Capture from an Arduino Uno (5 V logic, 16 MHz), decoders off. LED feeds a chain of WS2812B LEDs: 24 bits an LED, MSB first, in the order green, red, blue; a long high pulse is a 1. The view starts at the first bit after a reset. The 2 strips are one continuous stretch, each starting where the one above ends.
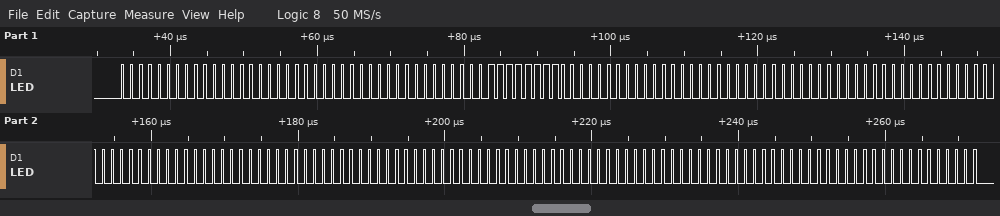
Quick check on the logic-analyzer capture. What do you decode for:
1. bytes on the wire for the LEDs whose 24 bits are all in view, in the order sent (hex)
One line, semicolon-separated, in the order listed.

00 00 00 00 00 FF 00 00 00 00 00 00 00 00 00 00 00 00 00 00 00 00 00 00
